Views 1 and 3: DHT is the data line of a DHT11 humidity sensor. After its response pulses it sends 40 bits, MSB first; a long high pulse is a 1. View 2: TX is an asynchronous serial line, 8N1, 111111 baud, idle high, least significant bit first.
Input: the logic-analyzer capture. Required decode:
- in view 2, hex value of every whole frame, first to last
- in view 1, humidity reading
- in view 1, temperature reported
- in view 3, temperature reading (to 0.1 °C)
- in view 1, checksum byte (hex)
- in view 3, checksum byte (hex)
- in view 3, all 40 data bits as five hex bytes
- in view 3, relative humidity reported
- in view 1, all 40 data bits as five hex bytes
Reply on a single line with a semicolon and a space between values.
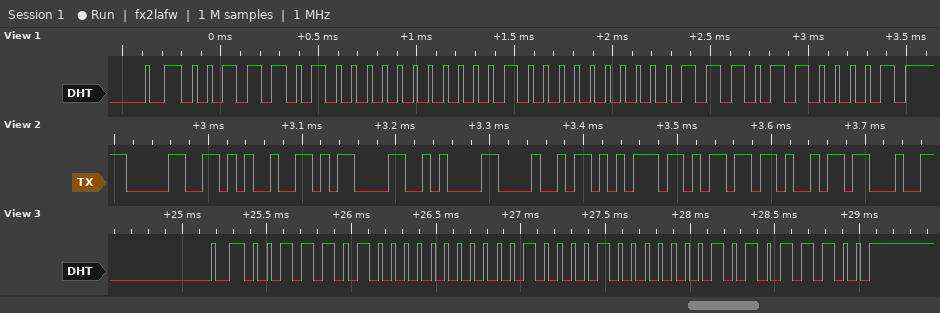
30 25 0D 0A 48 75 6D 69; 58 %; 32.7 °C; 33.1 °C; 0x61; 0x5C; 3A 00 21 01 5C; 58 %; 3A 00 20 07 61
